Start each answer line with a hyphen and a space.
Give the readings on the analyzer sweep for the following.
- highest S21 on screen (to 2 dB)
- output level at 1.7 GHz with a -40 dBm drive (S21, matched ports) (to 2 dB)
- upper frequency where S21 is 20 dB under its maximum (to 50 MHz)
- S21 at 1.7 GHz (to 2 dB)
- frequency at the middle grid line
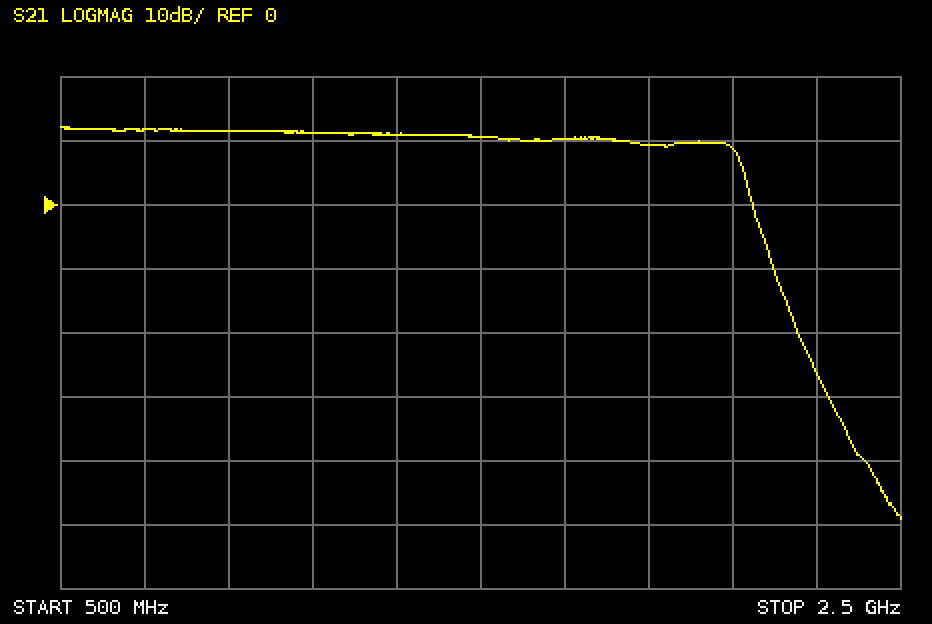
- 12 dB
- -30 dBm
- 2.20 GHz
- 10 dB
- 1.5 GHz
